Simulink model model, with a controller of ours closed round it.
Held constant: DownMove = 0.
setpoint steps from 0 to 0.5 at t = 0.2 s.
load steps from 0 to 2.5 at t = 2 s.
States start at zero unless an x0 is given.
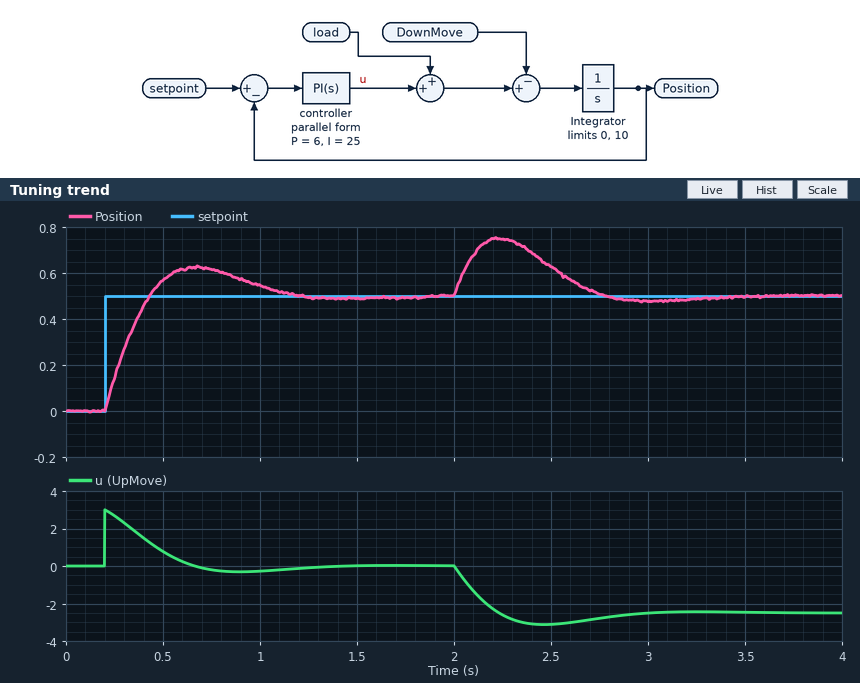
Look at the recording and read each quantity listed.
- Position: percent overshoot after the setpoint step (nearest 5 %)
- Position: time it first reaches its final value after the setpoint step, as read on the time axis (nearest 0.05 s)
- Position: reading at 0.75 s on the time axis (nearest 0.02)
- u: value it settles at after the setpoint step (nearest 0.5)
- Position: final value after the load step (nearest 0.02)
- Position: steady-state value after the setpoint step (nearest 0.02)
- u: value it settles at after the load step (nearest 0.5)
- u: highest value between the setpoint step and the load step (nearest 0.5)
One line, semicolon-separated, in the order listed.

25 %; 0.45 s; 0.62; 0.0; 0.50; 0.50; -2.5; 3.0
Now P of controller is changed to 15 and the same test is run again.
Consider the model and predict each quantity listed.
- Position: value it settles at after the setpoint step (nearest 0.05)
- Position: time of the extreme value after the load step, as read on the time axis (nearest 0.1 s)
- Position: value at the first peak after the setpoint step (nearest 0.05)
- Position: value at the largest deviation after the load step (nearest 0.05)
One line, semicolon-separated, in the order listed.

0.50; 2.2 s; 0.55; 0.65
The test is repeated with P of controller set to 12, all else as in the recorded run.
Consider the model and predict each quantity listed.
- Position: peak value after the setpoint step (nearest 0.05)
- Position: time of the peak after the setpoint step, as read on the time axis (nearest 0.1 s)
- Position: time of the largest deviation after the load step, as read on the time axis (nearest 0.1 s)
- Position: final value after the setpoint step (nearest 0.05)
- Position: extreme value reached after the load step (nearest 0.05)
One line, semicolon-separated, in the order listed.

0.55; 0.6 s; 2.2 s; 0.50; 0.65
